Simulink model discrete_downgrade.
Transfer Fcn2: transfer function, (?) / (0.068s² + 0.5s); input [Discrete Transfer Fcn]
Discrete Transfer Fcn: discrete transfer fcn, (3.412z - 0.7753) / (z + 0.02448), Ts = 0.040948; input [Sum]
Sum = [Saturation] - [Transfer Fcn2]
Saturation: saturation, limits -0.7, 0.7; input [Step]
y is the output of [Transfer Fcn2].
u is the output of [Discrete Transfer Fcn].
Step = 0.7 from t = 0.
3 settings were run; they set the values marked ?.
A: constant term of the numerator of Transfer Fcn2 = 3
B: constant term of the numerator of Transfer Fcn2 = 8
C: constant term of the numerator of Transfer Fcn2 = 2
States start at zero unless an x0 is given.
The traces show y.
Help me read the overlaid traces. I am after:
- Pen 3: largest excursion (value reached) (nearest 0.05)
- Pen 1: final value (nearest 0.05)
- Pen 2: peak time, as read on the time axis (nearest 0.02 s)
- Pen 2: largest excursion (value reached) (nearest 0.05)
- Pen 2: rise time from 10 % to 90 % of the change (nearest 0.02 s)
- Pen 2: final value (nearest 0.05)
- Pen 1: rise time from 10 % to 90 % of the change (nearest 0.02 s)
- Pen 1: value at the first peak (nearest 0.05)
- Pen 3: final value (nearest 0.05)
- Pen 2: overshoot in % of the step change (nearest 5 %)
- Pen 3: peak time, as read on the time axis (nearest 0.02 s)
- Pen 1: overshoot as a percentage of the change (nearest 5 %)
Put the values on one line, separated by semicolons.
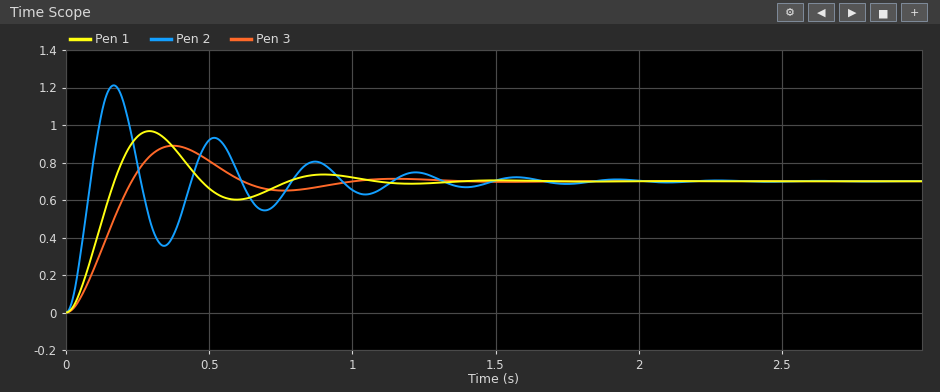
0.90; 0.70; 0.16 s; 1.20; 0.06 s; 0.70; 0.12 s; 0.95; 0.70; 75 %; 0.38 s; 40 %
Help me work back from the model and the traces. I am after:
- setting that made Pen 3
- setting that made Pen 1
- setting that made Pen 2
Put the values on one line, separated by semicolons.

C; A; B
